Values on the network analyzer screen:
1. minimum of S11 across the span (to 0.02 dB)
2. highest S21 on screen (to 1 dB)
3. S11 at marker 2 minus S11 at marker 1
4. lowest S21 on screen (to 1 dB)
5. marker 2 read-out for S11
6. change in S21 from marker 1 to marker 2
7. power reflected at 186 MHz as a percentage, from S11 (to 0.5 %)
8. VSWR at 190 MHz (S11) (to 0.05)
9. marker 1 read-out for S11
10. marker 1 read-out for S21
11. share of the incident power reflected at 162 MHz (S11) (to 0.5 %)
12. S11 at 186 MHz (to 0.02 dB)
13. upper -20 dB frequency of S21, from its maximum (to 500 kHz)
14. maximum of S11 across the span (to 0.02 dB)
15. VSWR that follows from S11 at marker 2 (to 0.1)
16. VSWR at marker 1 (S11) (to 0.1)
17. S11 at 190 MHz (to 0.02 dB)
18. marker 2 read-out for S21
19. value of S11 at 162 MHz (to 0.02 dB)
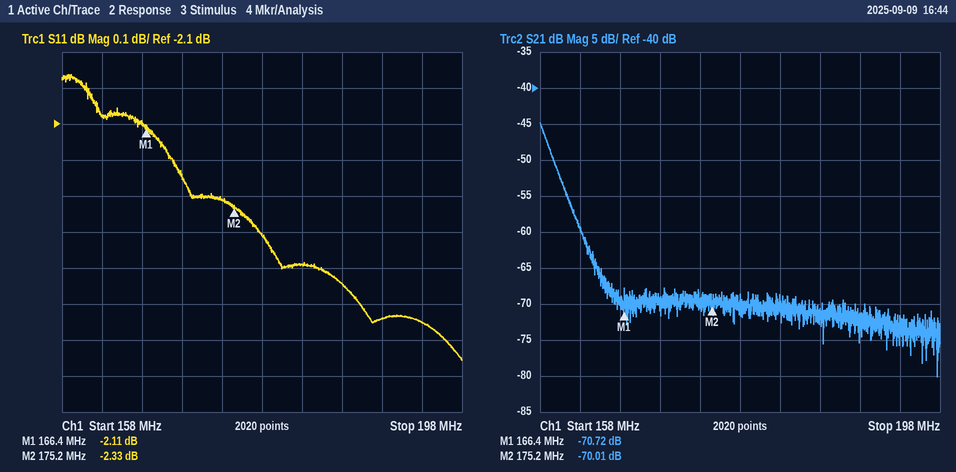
-2.76 dB
-45 dB
-0.22 dB
-80 dB
-2.33 dB
0.71 dB
55.5 %
6.65
-2.11 dB
-70.72 dB
62.0 %
-2.54 dB
163.5 MHz
-1.96 dB
7.5
8.3
-2.64 dB
-70.01 dB
-2.08 dB
